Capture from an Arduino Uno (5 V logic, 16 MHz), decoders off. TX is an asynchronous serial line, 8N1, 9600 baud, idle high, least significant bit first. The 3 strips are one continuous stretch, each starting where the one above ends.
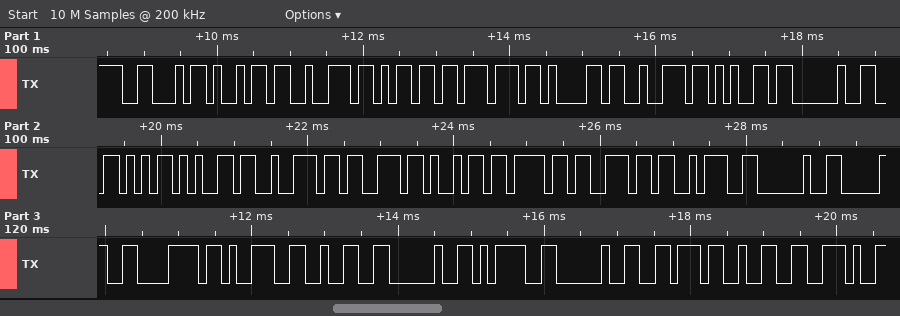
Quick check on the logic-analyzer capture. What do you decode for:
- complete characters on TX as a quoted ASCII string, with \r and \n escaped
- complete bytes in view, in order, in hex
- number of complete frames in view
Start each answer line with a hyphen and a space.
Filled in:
- "Firmware Version: 0x92 = v2."
- 0x46 0x69 0x72 0x6D 0x77 0x61 0x72 0x65 0x20 0x56 0x65 0x72 0x73 0x69 0x6F 0x6E 0x3A 0x20 0x30 0x78 0x39 0x32 0x20 0x3D 0x20 0x76 0x32 0x2E
- 28
